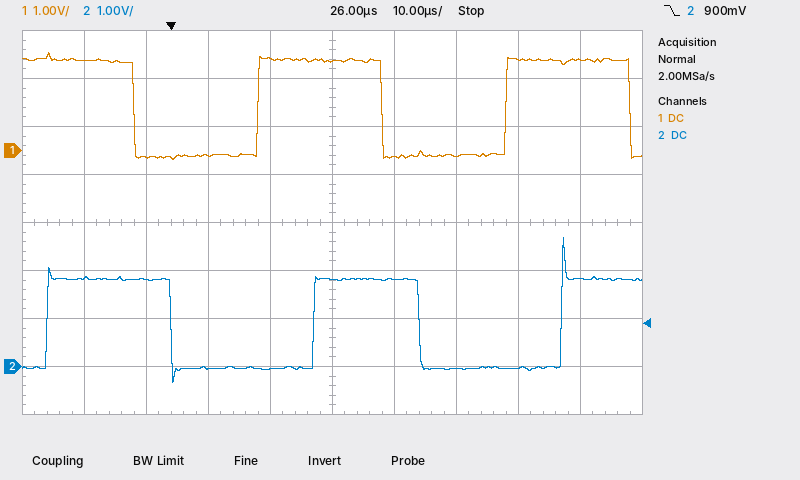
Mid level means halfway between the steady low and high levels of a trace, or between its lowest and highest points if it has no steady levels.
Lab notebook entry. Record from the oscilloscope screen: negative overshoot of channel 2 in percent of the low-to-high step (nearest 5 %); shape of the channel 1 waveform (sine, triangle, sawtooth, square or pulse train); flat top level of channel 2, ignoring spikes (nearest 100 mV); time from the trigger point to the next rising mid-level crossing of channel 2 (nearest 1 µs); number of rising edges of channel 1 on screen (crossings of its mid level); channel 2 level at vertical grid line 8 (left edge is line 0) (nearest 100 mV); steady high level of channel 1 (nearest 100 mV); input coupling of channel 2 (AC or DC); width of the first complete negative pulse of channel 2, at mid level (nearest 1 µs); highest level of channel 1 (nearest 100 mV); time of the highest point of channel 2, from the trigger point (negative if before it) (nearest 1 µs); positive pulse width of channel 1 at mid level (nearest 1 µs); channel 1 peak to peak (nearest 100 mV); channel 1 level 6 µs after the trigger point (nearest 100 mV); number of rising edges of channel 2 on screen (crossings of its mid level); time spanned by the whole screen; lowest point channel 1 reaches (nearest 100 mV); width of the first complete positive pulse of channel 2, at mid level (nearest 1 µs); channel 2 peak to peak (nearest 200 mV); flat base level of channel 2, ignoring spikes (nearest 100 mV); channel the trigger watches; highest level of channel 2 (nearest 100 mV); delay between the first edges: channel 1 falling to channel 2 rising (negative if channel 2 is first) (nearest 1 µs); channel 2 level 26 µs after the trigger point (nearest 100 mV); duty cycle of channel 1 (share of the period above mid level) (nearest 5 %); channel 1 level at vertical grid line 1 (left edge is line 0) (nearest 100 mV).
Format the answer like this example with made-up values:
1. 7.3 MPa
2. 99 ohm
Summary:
1. 15 %
2. square
3. 1.8 V
4. 23 µs
5. 2
6. 0.0 V
7. 1.9 V
8. DC
9. 23 µs
10. 2.0 V
11. +63 µs
12. 20 µs
13. 2.2 V
14. -100 mV
15. 3
16. 100 µs
17. -200 mV
18. 20 µs
19. 3.0 V
20. 0.0 V
21. channel 2
22. 2.7 V
23. -14 µs
24. 1.8 V
25. 50 %
26. 1.9 V
